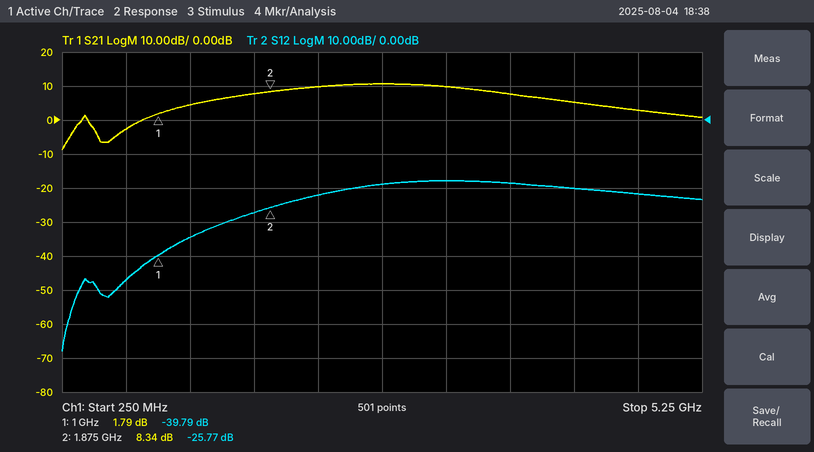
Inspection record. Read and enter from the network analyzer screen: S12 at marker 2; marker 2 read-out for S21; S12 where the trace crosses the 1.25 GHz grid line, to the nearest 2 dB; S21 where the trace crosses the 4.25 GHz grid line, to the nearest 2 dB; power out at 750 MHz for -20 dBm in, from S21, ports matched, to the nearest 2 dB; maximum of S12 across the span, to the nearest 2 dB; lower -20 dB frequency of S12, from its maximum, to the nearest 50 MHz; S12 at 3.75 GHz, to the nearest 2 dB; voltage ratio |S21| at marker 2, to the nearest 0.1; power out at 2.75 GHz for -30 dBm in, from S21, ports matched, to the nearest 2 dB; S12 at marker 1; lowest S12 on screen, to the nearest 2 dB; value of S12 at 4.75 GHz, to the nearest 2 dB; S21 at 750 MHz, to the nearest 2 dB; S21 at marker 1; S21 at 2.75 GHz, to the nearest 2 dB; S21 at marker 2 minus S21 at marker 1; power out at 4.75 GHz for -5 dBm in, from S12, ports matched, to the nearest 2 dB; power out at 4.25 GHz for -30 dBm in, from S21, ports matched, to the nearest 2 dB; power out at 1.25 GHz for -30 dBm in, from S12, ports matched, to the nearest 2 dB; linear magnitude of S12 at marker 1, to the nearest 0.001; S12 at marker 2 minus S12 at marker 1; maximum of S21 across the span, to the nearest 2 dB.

-25.77 dB
8.34 dB
-34 dB
6 dB
-22 dBm
-18 dB
1.10 GHz
-18 dB
2.6
-20 dBm
-39.79 dB
-68 dB
-22 dB
-2 dB
1.79 dB
10 dB
6.55 dB
-26 dBm
-24 dBm
-64 dBm
0.010
14.02 dB
10 dB
